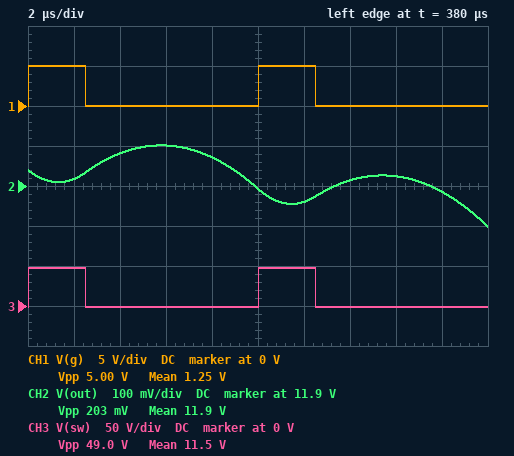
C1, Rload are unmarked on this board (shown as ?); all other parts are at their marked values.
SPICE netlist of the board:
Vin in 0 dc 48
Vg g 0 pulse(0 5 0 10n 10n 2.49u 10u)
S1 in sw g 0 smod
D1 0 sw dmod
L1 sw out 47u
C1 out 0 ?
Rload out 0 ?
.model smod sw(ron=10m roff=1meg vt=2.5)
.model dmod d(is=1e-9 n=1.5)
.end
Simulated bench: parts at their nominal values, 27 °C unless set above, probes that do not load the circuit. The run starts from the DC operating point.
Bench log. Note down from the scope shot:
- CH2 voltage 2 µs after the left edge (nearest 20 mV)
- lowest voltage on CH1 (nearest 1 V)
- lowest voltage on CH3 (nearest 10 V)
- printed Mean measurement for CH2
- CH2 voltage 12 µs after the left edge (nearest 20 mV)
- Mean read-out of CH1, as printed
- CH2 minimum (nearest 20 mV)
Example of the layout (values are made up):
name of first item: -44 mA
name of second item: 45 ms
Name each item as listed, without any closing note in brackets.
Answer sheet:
CH2 voltage 2 µs after the left edge: 11.92 V
lowest voltage on CH1: 0 V
lowest voltage on CH3: 0 V
printed Mean measurement for CH2: 11.9 V
CH2 voltage 12 µs after the left edge: 11.86 V
Mean read-out of CH1, as printed: 1.25 V
CH2 minimum: 11.80 V
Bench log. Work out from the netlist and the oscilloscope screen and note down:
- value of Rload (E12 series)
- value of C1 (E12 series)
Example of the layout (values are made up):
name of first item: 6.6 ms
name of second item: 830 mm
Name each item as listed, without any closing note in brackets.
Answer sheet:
value of Rload: 6.8 Ω
value of C1: 22 µF
